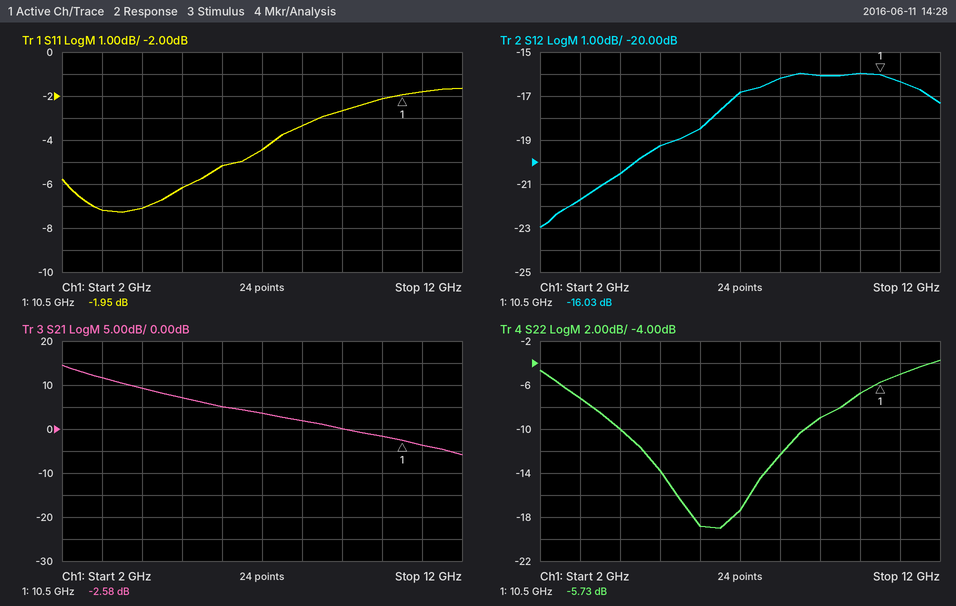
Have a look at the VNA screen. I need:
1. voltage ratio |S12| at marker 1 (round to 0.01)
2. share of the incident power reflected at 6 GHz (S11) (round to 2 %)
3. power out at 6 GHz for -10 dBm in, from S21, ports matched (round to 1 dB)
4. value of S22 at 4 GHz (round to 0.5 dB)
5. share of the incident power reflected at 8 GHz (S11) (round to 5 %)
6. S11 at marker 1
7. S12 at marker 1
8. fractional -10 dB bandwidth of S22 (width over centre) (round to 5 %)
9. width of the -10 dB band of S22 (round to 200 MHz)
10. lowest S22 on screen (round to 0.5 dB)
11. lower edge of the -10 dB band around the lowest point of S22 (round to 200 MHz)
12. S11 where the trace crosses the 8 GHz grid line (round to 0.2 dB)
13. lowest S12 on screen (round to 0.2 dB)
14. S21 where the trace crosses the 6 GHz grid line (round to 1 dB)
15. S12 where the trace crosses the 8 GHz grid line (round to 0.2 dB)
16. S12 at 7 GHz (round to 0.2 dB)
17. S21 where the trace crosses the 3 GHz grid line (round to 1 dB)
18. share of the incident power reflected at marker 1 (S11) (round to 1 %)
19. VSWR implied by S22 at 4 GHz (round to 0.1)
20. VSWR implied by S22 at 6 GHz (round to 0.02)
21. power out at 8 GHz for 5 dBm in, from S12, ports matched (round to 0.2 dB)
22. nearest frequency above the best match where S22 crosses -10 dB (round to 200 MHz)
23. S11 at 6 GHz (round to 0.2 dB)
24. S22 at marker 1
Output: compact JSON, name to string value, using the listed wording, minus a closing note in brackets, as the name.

{"voltage ratio |S12| at marker 1": "0.16", "share of the incident power reflected at 6 GHz (S11)": "30 %", "power out at 6 GHz for -10 dBm in, from S21, ports matched": "-5 dBm", "value of S22 at 4 GHz": "-10.0 dB", "share of the incident power reflected at 8 GHz (S11)": "45 %", "S11 at marker 1": "-1.95 dB", "S12 at marker 1": "-16.03 dB", "fractional -10 dB bandwidth of S22 (width over centre)": "75 %", "width of the -10 dB band of S22": "4.6 GHz", "lowest S22 on screen": "-19.0 dB", "lower edge of the -10 dB band around the lowest point of S22": "4.0 GHz", "S11 where the trace crosses the 8 GHz grid line": "-3.4 dB", "lowest S12 on screen": "-23.0 dB", "S21 where the trace crosses the 6 GHz grid line": "5 dB", "S12 where the trace crosses the 8 GHz grid line": "-16.2 dB", "S12 at 7 GHz": "-16.8 dB", "S21 where the trace crosses the 3 GHz grid line": "12 dB", "share of the incident power reflected at marker 1 (S11)": "64 %", "VSWR implied by S22 at 4 GHz": "1.9", "VSWR implied by S22 at 6 GHz": "1.26", "power out at 8 GHz for 5 dBm in, from S12, ports matched": "-11.2 dBm", "nearest frequency above the best match where S22 crosses -10 dB": "8.6 GHz", "S11 at 6 GHz": "-5.2 dB", "S22 at marker 1": "-5.73 dB"}
